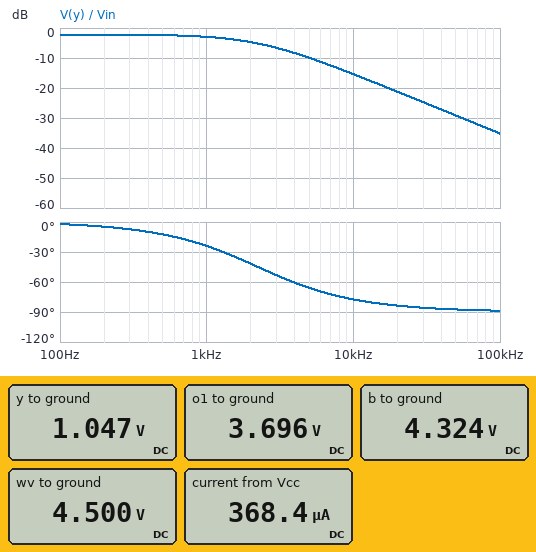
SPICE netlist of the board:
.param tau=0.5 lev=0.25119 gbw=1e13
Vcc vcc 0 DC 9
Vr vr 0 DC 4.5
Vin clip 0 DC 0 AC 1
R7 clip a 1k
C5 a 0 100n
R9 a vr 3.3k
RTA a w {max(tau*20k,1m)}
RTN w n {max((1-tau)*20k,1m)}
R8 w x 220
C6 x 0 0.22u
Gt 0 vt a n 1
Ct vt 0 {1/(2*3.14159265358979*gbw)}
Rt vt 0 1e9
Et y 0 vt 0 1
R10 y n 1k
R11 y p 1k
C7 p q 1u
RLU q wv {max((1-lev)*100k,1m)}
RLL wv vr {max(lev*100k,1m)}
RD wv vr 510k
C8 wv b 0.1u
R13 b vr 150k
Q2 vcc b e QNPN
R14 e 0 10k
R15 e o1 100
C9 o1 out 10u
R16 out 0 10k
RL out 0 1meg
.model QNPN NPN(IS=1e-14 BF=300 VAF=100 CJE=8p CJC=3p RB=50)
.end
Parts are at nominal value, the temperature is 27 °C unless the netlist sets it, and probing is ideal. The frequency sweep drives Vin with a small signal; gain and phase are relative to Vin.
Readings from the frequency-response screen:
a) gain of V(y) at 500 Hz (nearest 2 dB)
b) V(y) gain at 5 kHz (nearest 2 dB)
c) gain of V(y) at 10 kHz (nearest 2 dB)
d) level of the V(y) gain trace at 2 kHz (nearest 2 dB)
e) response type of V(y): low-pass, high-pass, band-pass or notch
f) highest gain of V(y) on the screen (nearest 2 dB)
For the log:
-2 dB
-10 dB
-16 dB
-4 dB
low-pass
-2 dB
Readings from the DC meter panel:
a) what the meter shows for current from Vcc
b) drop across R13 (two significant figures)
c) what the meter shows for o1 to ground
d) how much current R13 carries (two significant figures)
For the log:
368.4 µA
180 mV
3.696 V
1.2 µA
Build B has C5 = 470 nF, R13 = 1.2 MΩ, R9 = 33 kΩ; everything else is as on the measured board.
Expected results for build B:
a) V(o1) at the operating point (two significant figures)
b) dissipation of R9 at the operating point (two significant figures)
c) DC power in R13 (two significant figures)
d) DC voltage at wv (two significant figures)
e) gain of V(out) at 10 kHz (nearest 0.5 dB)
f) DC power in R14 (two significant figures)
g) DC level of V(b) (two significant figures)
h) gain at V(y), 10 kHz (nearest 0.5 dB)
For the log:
2.8 V
580 µW
940 nW
4.5 V
-41.5 dB
790 µW
3.4 V
-28.5 dB
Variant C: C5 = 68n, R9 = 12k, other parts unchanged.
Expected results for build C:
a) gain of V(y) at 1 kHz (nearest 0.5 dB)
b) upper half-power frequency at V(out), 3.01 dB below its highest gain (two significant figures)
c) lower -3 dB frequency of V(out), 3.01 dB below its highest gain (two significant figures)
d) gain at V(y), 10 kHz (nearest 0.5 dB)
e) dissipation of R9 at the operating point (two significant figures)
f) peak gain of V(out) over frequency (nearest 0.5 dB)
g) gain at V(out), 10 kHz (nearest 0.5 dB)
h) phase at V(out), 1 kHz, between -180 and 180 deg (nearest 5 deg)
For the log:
-1.0 dB
2.8 kHz
11 Hz
-12.0 dB
1.4 mW
-14.5 dB
-26.0 dB
-20 deg
